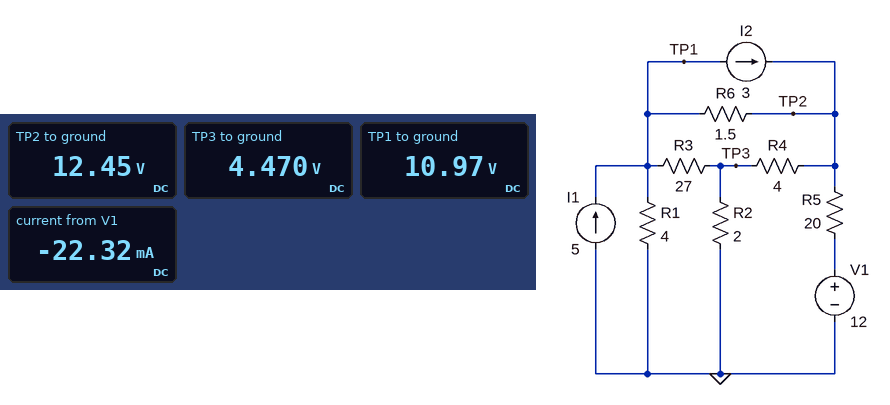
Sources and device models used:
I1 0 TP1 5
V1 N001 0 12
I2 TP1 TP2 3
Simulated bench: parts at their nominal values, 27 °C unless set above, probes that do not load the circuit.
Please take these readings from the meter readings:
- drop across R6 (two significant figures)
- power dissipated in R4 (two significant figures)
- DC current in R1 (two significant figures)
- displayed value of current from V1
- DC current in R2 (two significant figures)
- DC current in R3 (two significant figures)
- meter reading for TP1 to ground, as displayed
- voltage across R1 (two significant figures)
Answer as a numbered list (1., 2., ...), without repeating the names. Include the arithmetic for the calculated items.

1. 12.45 V - 10.97 V = 1.5 V
2. (12.45 V - 4.47 V)^2 / 4 Ω = 16 W
3. (10.97 V) / 4 Ω = 2.7 A
4. -22.32 mA
5. (4.47 V) / 2 Ω = 2.2 A
6. (10.97 V - 4.47 V) / 27 Ω = 240 mA
7. 10.97 V
8. 10.97 V = 11 V
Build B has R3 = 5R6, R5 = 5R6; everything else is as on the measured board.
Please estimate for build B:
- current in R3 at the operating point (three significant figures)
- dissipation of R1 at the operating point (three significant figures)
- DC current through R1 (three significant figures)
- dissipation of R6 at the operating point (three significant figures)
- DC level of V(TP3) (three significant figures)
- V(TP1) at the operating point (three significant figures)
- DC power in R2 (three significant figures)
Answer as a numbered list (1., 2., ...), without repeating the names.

1. 855 mA
2. 24.4 W
3. 2.47 A
4. 2.64 W
5. 5.10 V
6. 9.89 V
7. 13.0 W
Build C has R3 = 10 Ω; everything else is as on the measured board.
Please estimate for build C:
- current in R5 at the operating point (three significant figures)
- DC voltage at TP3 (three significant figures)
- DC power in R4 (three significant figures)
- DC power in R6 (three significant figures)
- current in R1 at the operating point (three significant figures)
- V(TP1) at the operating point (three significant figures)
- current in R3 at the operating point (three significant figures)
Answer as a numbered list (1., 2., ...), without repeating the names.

1. 6.53 mA
2. 4.79 V
3. 13.5 W
4. 2.01 W
5. 2.60 A
6. 10.4 V
7. 560 mA
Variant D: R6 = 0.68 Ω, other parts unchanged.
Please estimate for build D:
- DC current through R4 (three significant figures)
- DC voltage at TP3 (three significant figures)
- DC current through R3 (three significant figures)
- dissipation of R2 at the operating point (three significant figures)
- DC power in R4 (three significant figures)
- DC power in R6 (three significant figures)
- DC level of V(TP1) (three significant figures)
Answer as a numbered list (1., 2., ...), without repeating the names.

1. 1.92 A
2. 4.35 V
3. 257 mA
4. 9.47 W
5. 14.7 W
6. 793 mW
7. 11.3 V
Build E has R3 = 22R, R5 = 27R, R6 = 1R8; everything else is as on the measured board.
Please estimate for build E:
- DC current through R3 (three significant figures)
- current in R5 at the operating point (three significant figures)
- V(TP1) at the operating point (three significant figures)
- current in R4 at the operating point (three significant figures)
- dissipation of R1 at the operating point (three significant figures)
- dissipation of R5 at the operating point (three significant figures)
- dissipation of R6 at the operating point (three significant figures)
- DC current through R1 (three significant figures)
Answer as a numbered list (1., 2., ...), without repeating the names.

1. 283 mA
2. 20.6 mA
3. 10.8 V
4. 2.00 A
5. 29.1 W
6. 11.5 mW
7. 1.73 W
8. 2.70 A
